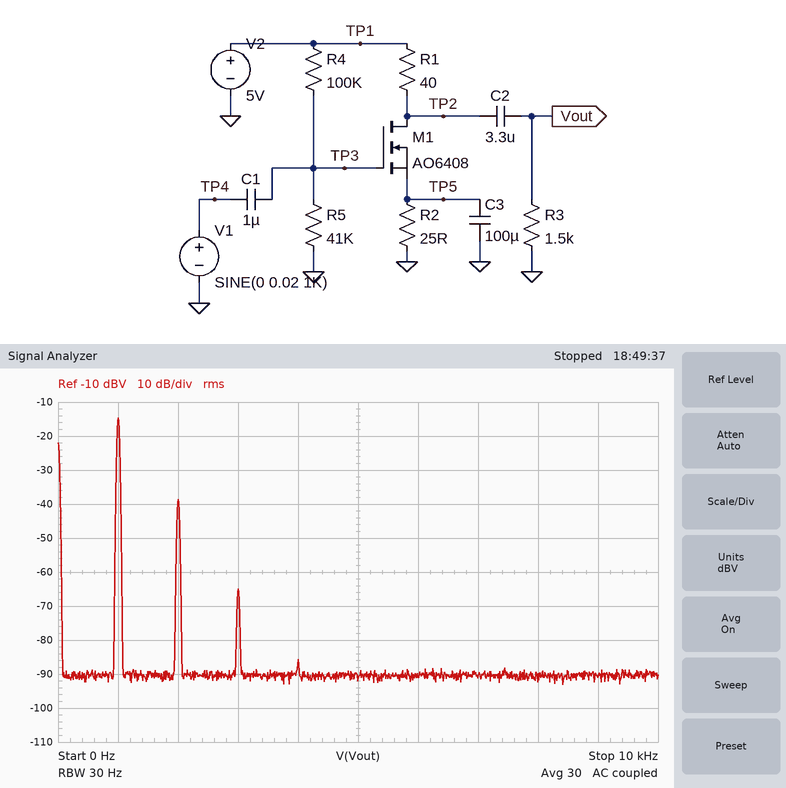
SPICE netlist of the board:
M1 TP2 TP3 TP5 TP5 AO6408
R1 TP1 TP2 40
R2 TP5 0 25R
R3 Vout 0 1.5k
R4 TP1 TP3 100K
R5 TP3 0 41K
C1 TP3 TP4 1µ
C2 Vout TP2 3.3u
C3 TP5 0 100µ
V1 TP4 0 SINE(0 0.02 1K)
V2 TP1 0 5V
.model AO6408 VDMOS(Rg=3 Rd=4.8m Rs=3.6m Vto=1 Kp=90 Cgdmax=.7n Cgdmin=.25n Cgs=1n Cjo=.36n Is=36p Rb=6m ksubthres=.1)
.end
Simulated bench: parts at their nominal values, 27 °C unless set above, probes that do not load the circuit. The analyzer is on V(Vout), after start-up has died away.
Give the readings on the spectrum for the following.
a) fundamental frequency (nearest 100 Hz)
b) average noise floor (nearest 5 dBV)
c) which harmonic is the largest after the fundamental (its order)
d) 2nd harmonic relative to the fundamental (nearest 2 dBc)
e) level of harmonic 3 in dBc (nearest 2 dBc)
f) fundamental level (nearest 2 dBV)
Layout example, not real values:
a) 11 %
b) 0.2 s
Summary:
a) 1.0 kHz
b) -90 dBV
c) 2
d) -24 dBc
e) -50 dBc
f) -14 dBV
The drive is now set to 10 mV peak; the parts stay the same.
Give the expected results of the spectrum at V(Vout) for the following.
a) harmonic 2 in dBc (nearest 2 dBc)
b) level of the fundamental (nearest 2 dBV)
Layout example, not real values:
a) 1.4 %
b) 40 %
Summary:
a) -30 dBc
b) -20 dBV
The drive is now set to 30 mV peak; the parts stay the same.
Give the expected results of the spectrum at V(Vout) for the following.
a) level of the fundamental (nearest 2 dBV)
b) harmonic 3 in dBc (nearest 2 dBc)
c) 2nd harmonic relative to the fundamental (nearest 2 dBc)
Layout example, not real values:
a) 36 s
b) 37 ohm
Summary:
a) -12 dBV
b) -44 dBc
c) -20 dBc
